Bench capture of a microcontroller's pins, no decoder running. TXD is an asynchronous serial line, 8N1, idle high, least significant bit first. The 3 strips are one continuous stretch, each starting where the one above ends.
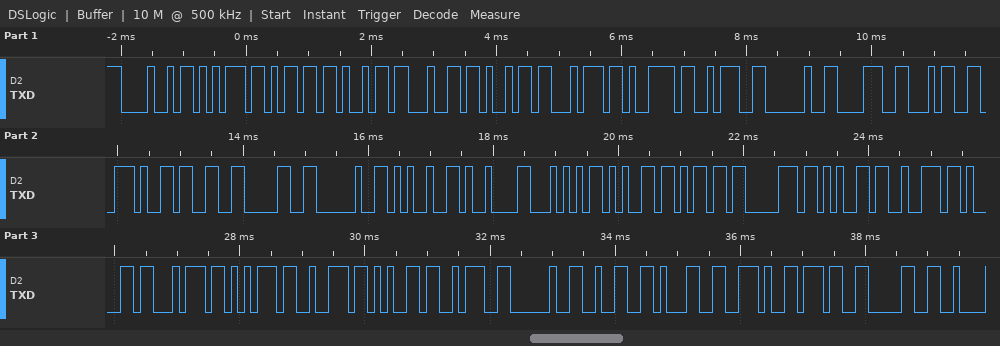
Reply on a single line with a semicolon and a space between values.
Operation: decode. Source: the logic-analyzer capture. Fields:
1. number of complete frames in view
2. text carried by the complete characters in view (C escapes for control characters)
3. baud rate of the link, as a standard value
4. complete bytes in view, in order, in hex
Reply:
36; "Humidity: 84.30 %\tTemperature: 21.70"; 9600 baud; 0x48 0x75 0x6D 0x69 0x64 0x69 0x74 0x79 0x3A 0x20 0x38 0x34 0x2E 0x33 0x30 0x20 0x25 0x09 0x54 0x65 0x6D 0x70 0x65 0x72 0x61 0x74 0x75 0x72 0x65 0x3A 0x20 0x32 0x31 0x2E 0x37 0x30
